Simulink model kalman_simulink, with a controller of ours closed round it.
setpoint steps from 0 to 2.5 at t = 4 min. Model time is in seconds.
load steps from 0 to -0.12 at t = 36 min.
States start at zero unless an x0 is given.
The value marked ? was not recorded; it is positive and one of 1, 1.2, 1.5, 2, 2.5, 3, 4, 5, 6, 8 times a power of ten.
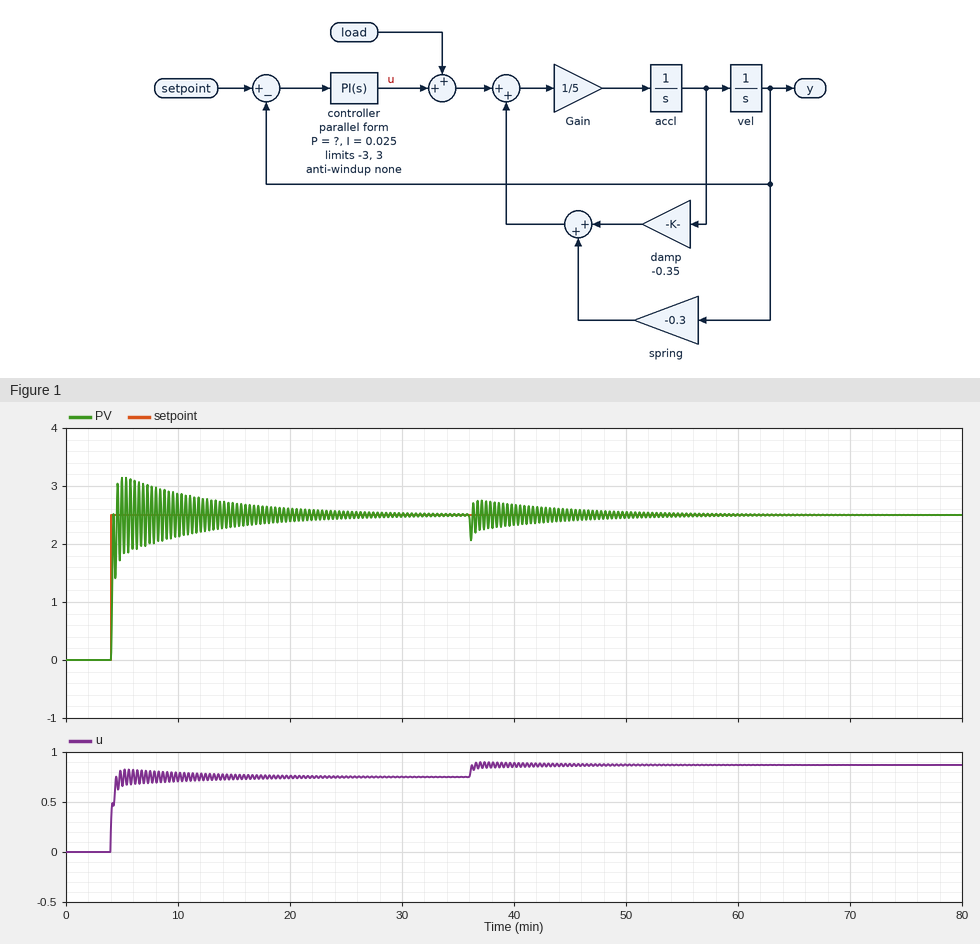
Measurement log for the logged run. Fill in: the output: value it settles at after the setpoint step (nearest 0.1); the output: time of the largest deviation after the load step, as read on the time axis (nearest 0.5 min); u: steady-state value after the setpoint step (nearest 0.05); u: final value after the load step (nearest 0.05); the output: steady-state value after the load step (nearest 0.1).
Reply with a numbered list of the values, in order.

1. 2.5
2. 36.0 min
3. 0.75
4. 0.85
5. 2.5
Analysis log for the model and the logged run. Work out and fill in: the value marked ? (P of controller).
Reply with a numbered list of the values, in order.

1. 0.08
